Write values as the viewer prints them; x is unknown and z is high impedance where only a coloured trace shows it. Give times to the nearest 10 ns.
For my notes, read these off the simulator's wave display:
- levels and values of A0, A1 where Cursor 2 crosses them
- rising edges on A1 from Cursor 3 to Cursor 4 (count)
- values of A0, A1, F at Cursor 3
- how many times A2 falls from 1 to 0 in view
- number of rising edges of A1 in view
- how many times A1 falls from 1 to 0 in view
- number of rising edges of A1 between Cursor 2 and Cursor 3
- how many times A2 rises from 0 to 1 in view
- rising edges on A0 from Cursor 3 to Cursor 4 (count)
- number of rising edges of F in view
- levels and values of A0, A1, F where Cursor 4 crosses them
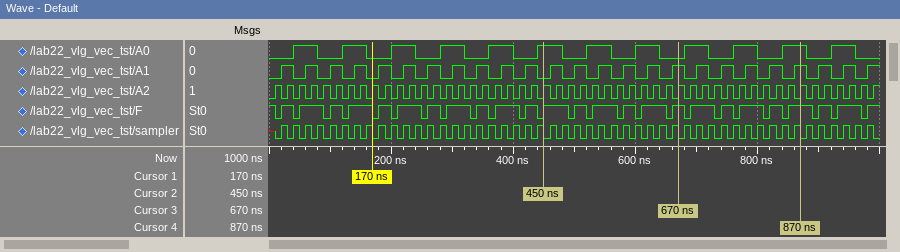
A0=1, A1=0
5
A0=0, A1=1, F=1
49
25
24
6
50
3
25
A0=1, A1=1, F=1
